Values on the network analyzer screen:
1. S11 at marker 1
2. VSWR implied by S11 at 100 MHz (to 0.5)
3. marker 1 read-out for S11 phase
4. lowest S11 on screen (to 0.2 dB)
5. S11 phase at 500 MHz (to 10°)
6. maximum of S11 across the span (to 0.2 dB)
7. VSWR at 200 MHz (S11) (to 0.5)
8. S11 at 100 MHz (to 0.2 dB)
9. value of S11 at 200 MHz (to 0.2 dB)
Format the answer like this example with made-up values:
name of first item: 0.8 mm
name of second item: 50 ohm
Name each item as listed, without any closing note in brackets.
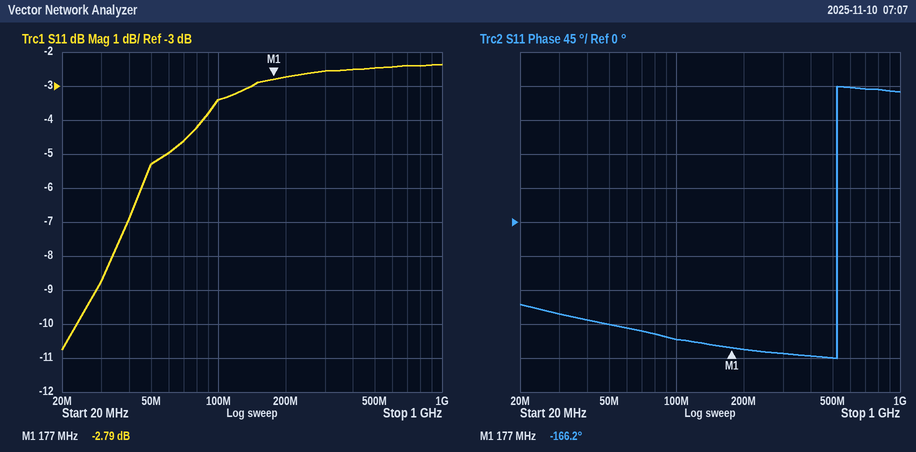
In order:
S11 at marker 1: -2.79 dB
VSWR implied by S11 at 100 MHz: 5.0
marker 1 read-out for S11 phase: -166.2°
lowest S11 on screen: -10.8 dB
S11 phase at 500 MHz: -180°
maximum of S11 across the span: -2.4 dB
VSWR at 200 MHz (S11): 6.5
S11 at 100 MHz: -3.4 dB
value of S11 at 200 MHz: -2.8 dB
